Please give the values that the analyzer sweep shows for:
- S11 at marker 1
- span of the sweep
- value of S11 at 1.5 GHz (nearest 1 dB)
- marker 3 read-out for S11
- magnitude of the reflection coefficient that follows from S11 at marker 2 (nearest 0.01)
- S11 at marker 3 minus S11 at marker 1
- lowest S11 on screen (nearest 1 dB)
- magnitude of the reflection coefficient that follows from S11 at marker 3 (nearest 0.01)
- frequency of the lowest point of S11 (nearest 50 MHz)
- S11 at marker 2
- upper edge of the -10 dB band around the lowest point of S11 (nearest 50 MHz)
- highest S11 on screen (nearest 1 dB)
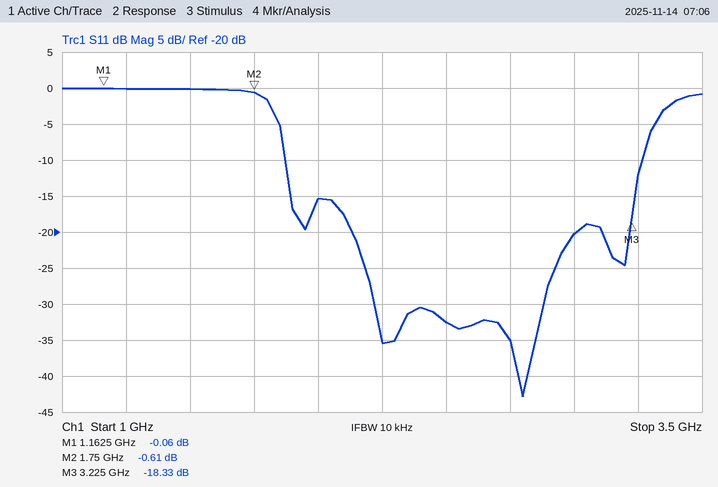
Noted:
-0.06 dB
2.5 GHz
0 dB
-18.33 dB
0.93
-18.27 dB
-43 dB
0.12
2.80 GHz
-0.61 dB
3.25 GHz
0 dB
